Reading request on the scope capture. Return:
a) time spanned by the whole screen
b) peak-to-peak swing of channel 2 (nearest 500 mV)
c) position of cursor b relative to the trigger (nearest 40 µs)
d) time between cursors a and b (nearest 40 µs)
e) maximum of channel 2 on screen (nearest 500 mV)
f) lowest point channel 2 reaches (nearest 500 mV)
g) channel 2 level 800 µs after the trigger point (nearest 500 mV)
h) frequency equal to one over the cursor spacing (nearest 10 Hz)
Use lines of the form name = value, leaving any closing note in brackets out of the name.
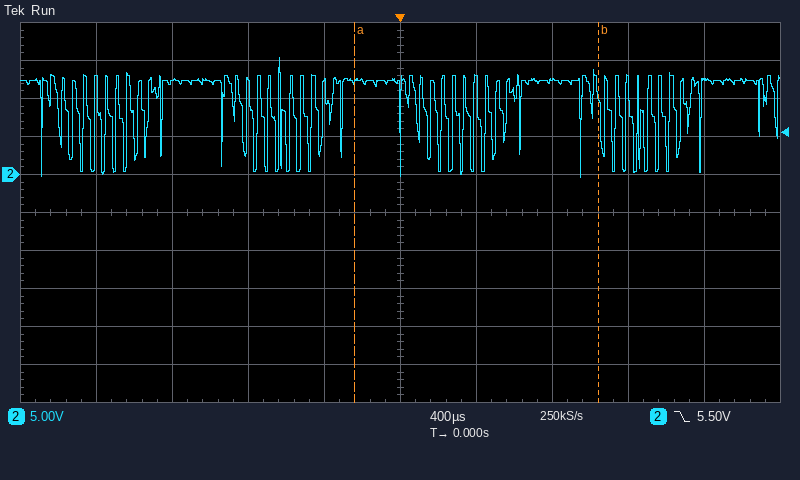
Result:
time spanned by the whole screen = 4 ms
peak-to-peak swing of channel 2 = 16.0 V
position of cursor b relative to the trigger = +1.04 ms
time between cursors a and b = 1.28 ms
maximum of channel 2 on screen = 15.5 V
lowest point channel 2 reaches = -500 mV
channel 2 level 800 µs after the trigger point = 12.5 V
frequency equal to one over the cursor spacing = 780 Hz
